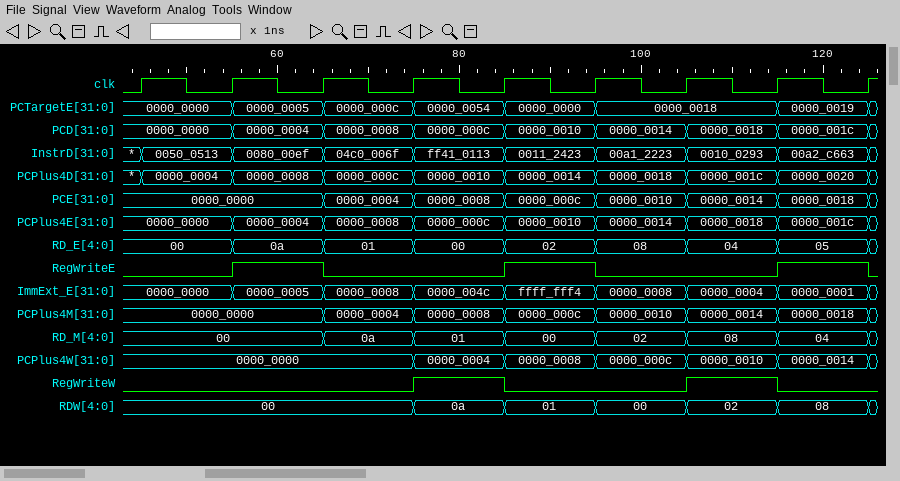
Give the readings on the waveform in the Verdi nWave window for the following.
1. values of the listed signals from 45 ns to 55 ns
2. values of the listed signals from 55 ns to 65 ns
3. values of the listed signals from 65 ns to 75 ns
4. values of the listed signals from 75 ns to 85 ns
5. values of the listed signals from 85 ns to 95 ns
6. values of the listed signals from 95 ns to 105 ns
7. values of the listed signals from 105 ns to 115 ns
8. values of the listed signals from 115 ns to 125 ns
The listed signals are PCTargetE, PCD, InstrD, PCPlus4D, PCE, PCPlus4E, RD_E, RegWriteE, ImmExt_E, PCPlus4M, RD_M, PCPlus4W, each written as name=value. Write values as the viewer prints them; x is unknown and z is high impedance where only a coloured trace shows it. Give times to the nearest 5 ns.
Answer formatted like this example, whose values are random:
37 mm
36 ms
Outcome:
PCTargetE=0000_0000, PCD=0000_0000, InstrD=0050_0513, PCPlus4D=0000_0004, PCE=0000_0000, PCPlus4E=0000_0000, RD_E=00, RegWriteE=0, ImmExt_E=0000_0000, PCPlus4M=0000_0000, RD_M=00, PCPlus4W=0000_0000
PCTargetE=0000_0005, PCD=0000_0004, InstrD=0080_00ef, PCPlus4D=0000_0008, PCE=0000_0000, PCPlus4E=0000_0004, RD_E=0a, RegWriteE=1, ImmExt_E=0000_0005, PCPlus4M=0000_0000, RD_M=00, PCPlus4W=0000_0000
PCTargetE=0000_000c, PCD=0000_0008, InstrD=04c0_006f, PCPlus4D=0000_000c, PCE=0000_0004, PCPlus4E=0000_0008, RD_E=01, RegWriteE=0, ImmExt_E=0000_0008, PCPlus4M=0000_0004, RD_M=0a, PCPlus4W=0000_0000
PCTargetE=0000_0054, PCD=0000_000c, InstrD=ff41_0113, PCPlus4D=0000_0010, PCE=0000_0008, PCPlus4E=0000_000c, RD_E=00, RegWriteE=0, ImmExt_E=0000_004c, PCPlus4M=0000_0008, RD_M=01, PCPlus4W=0000_0004
PCTargetE=0000_0000, PCD=0000_0010, InstrD=0011_2423, PCPlus4D=0000_0014, PCE=0000_000c, PCPlus4E=0000_0010, RD_E=02, RegWriteE=1, ImmExt_E=ffff_fff4, PCPlus4M=0000_000c, RD_M=00, PCPlus4W=0000_0008
PCTargetE=0000_0018, PCD=0000_0014, InstrD=00a1_2223, PCPlus4D=0000_0018, PCE=0000_0010, PCPlus4E=0000_0014, RD_E=08, RegWriteE=0, ImmExt_E=0000_0008, PCPlus4M=0000_0010, RD_M=02, PCPlus4W=0000_000c
PCTargetE=0000_0018, PCD=0000_0018, InstrD=0010_0293, PCPlus4D=0000_001c, PCE=0000_0014, PCPlus4E=0000_0018, RD_E=04, RegWriteE=0, ImmExt_E=0000_0004, PCPlus4M=0000_0014, RD_M=08, PCPlus4W=0000_0010
PCTargetE=0000_0019, PCD=0000_001c, InstrD=00a2_c663, PCPlus4D=0000_0020, PCE=0000_0018, PCPlus4E=0000_001c, RD_E=05, RegWriteE=1, ImmExt_E=0000_0001, PCPlus4M=0000_0018, RD_M=04, PCPlus4W=0000_0014
